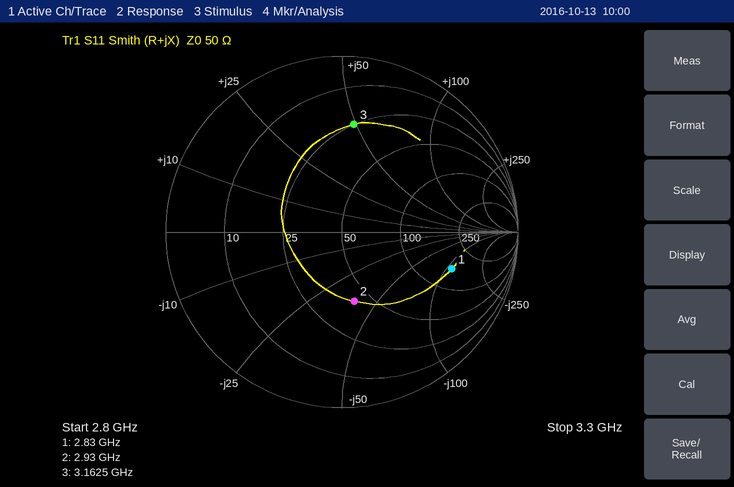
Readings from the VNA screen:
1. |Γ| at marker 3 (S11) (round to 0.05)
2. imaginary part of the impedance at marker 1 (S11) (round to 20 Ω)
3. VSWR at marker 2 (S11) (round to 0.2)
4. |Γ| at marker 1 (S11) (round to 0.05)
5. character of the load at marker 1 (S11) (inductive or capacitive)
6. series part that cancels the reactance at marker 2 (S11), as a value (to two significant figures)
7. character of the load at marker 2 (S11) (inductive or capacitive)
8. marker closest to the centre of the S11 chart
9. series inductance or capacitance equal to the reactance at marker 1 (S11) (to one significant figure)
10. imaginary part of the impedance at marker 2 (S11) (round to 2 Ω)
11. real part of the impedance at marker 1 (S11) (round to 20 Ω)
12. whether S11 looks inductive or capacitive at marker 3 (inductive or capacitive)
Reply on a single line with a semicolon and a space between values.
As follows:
0.60; -120 Ω; 2.4; 0.65; capacitive; 2.1 nH; capacitive; marker 2; 500 fF; -38 Ω; 160 Ω; inductive
